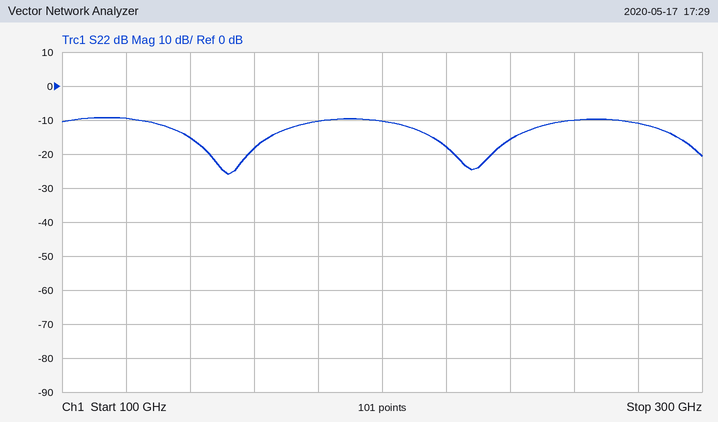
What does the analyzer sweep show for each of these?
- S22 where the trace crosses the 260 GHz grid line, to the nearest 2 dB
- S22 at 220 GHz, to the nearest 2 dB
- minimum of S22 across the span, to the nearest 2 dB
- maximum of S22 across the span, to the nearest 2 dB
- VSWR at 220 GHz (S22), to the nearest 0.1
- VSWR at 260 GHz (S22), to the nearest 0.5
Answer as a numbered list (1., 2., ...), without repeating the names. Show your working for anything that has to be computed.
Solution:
1. -10 dB
2. -18 dB
3. -26 dB
4. -10 dB
5. |Γ| = 10^(-18/20) = 0.1259; VSWR = (1 + 0.1259)/(1 − 0.1259) ≈ 1.3
6. |Γ| = 10^(-10/20) = 0.3162; VSWR = (1 + 0.3162)/(1 − 0.3162) ≈ 1.92, so 2.0 to the nearest 0.5
